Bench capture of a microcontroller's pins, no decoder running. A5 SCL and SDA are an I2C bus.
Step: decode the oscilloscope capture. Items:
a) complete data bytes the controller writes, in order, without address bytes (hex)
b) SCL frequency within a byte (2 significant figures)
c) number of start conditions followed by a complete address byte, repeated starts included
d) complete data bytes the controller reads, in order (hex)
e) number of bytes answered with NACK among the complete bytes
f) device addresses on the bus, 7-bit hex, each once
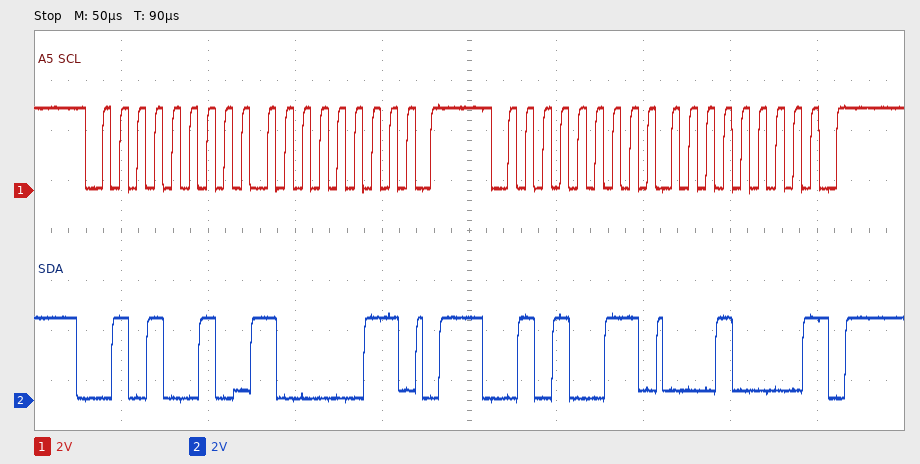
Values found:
83
100 kHz
2
10
1
0x29
